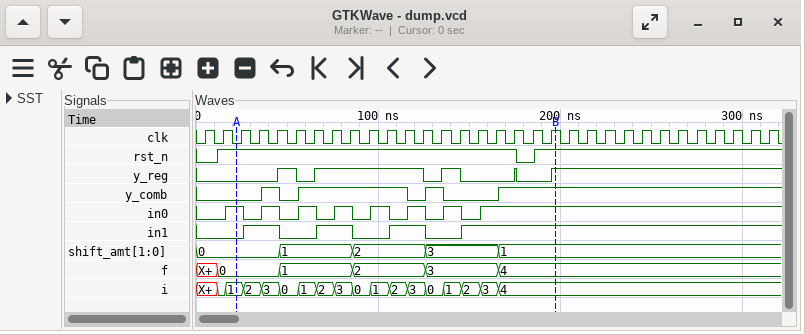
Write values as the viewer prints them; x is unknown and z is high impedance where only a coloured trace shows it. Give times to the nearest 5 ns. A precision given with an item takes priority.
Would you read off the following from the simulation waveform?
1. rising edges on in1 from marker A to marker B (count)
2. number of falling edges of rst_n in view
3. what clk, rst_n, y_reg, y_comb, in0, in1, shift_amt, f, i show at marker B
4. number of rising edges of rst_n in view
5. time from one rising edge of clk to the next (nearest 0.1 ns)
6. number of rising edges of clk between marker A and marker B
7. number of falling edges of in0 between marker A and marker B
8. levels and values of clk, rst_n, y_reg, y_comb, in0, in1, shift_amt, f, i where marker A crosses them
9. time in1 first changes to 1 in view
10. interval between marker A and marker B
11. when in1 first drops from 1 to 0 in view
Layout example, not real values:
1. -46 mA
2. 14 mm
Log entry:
1. 4
2. 1
3. clk=1, rst_n=1, y_reg=1, y_comb=1, in0=1, in1=1, shift_amt=1, f=4, i=4
4. 2
5. 10 ns
6. 18
7. 7
8. clk=0, rst_n=1, y_reg=0, y_comb=0, in0=1, in1=0, shift_amt=0, f=0, i=1
9. 25 ns
10. 175 ns
11. 45 ns
